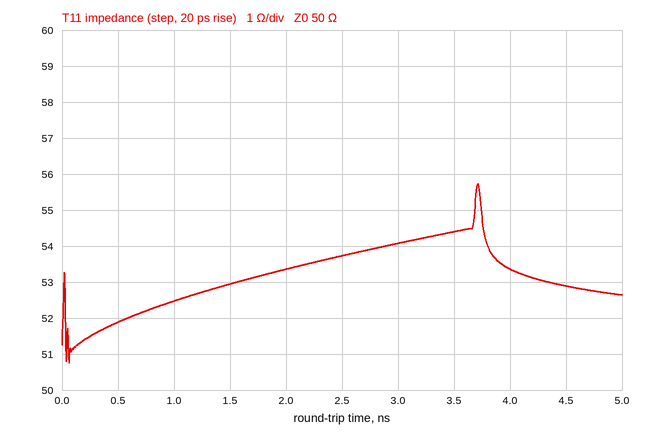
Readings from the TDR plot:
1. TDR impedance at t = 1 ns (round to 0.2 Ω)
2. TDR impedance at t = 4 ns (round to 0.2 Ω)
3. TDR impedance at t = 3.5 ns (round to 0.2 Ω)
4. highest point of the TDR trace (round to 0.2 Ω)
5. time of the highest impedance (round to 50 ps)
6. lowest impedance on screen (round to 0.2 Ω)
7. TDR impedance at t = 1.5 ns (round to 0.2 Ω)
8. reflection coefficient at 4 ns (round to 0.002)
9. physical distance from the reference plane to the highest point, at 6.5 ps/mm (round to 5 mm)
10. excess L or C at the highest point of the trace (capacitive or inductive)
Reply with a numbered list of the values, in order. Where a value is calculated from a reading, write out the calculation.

1. 52.4 Ω
2. 53.4 Ω
3. 54.4 Ω
4. 55.8 Ω
5. 3.70 ns
6. 50.8 Ω
7. 53.0 Ω
8. (53.4 − 50)/(53.4 + 50) ≈ +0.0329, so +0.032 to the nearest 0.002
9. 3.70 ns / 2 / 6.5 ps/mm ≈ 285 mm
10. inductive
